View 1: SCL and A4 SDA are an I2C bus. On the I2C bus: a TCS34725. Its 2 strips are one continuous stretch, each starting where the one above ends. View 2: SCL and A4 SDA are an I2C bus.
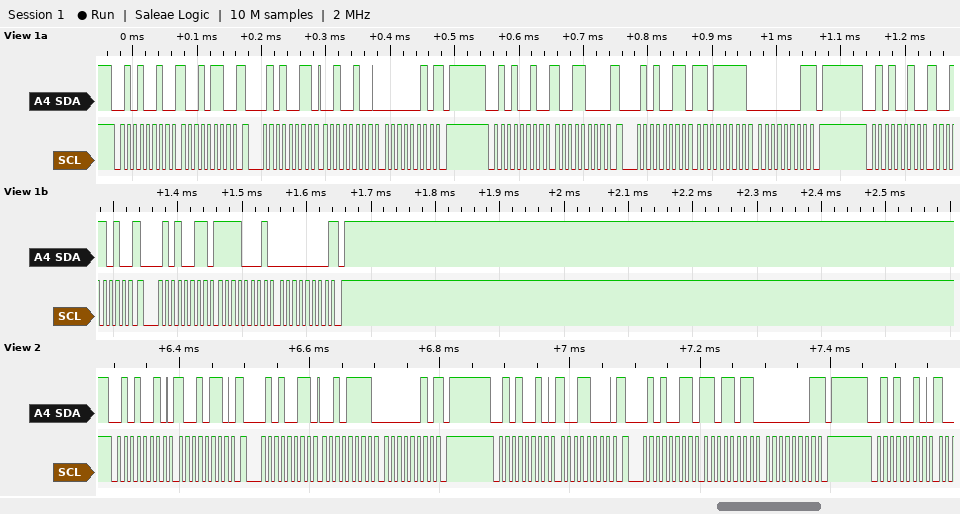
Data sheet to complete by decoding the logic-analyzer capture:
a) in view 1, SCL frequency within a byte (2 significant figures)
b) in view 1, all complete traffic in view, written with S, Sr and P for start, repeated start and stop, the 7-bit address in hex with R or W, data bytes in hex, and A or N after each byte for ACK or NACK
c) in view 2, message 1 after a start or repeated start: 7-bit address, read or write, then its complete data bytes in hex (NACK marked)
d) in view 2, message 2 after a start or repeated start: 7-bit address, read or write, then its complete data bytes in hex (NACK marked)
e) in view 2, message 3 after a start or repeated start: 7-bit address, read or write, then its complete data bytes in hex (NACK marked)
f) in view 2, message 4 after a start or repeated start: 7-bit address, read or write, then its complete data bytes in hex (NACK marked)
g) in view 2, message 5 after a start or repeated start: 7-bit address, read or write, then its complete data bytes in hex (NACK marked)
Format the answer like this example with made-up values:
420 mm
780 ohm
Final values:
100 kHz
S 29W A 96 A Sr 29R A 24 A 02 N P S 29W A 98 A Sr 29R A DF A 01 N P S 29W A 9A A Sr 29R A F1 A 00 N P
0x29 write: 96
0x29 read: 2F 02 NACK
0x29 write: 98
0x29 read: DB 01 NACK
0x29 write
